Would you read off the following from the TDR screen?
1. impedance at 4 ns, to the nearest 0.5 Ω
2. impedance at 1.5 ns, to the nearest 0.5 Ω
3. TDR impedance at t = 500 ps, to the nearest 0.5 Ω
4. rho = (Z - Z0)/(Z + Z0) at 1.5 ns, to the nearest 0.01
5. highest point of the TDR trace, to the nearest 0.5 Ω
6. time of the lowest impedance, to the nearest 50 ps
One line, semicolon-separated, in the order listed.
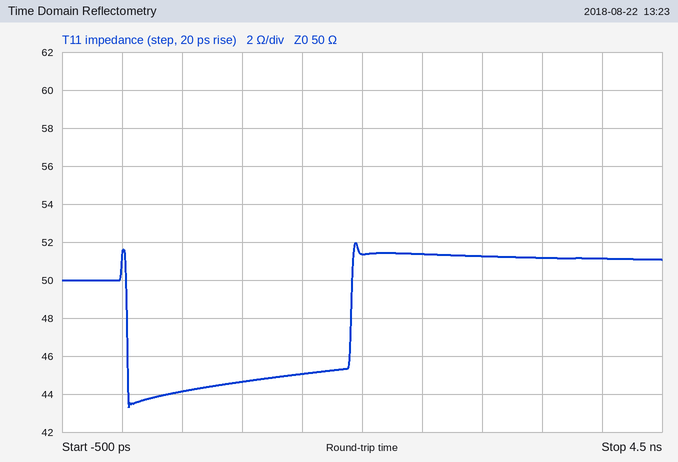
51.0 Ω; 45.0 Ω; 44.0 Ω; -0.05; 52.0 Ω; 50 ps
